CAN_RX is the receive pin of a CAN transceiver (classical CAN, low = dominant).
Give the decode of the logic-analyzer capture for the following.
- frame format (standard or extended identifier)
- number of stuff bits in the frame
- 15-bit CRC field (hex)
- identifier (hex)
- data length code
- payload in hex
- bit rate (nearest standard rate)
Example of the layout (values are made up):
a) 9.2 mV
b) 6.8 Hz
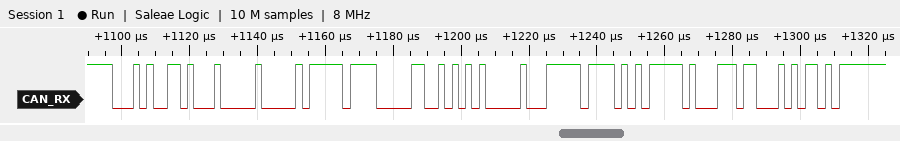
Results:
a) standard
b) 7
c) 0x6C56
d) 0x14D
e) 8
f) 00 FF 82 55 00 FF AB F1
g) 500 kbit/s
